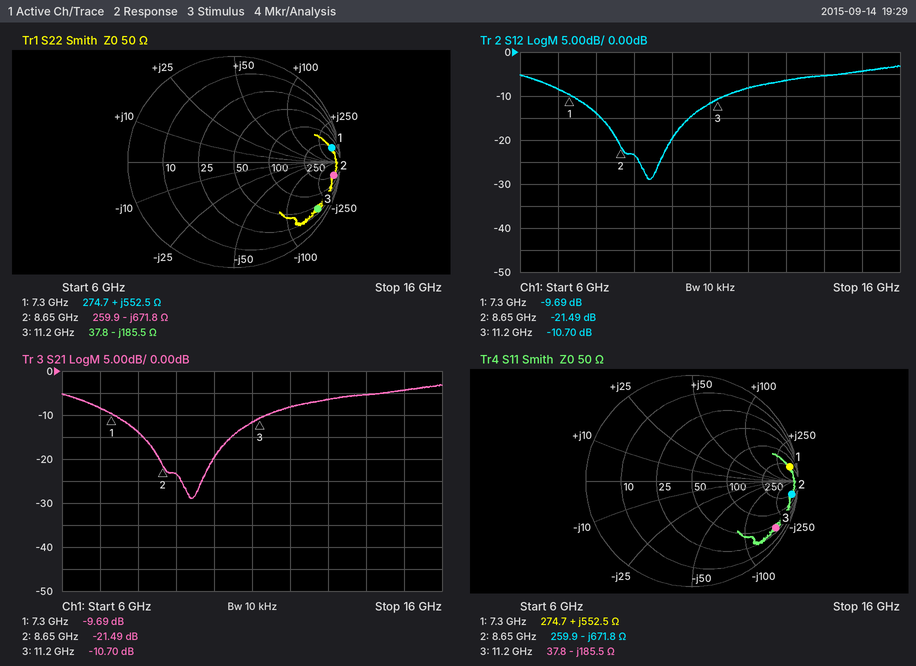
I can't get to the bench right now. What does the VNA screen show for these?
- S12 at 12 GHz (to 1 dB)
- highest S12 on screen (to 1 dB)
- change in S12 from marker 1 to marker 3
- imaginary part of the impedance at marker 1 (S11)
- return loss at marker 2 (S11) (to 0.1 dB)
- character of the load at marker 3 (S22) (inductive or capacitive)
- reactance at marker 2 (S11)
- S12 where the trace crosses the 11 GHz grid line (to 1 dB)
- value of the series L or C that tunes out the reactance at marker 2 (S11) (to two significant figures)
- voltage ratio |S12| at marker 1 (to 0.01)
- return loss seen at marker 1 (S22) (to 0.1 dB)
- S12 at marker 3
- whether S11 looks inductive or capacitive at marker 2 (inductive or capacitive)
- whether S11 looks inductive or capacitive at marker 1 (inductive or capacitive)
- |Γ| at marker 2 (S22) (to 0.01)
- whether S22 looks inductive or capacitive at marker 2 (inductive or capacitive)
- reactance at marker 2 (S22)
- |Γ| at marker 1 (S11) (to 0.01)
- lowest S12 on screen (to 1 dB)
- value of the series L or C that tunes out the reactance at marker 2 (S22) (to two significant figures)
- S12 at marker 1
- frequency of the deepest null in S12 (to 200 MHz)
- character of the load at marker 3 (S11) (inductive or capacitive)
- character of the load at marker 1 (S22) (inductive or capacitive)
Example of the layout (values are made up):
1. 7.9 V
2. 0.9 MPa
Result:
1. -8 dB
2. -3 dB
3. -1.01 dB
4. +552.5 Ω
5. 0.4 dB
6. capacitive
7. -671.8 Ω
8. -12 dB
9. 12 nH
10. 0.33
11. 0.6 dB
12. -10.70 dB
13. capacitive
14. inductive
15. 0.95
16. capacitive
17. -671.8 Ω
18. 0.93
19. -29 dB
20. 12 nH
21. -9.69 dB
22. 9.4 GHz
23. capacitive
24. inductive
